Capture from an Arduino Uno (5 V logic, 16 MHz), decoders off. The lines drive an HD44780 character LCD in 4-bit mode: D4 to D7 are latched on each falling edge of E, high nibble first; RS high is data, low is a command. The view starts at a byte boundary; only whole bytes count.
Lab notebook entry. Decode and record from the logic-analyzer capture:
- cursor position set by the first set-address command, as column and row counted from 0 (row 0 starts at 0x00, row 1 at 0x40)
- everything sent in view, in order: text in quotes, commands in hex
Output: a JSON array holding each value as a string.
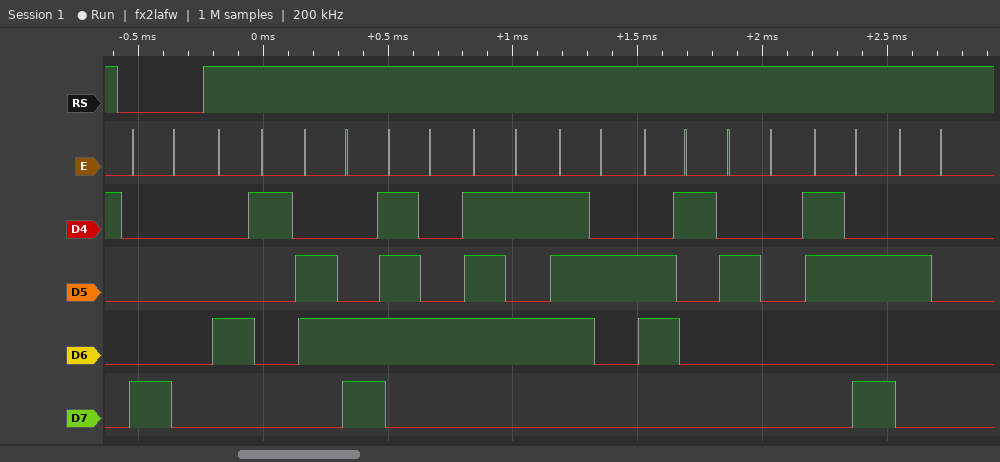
["column 0, row 0", "0x80 \"Altura : \""]
